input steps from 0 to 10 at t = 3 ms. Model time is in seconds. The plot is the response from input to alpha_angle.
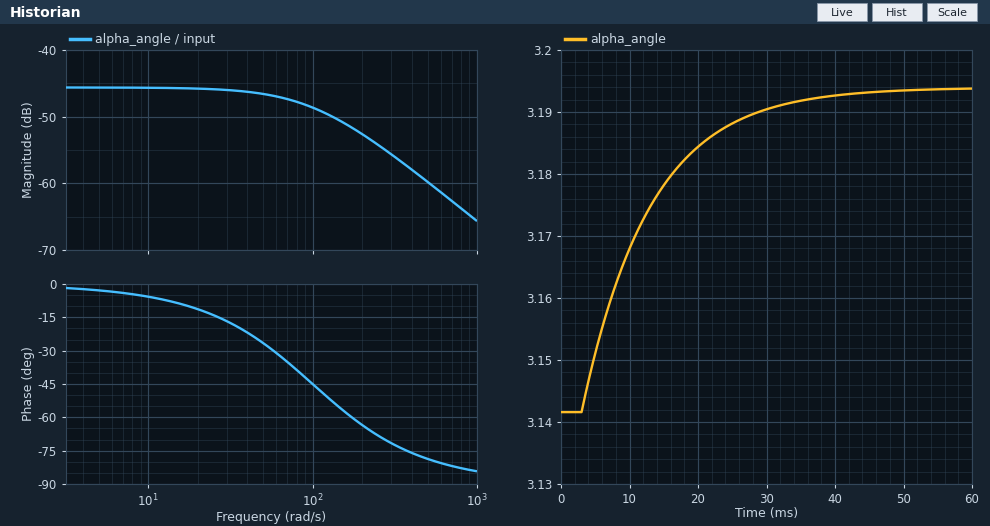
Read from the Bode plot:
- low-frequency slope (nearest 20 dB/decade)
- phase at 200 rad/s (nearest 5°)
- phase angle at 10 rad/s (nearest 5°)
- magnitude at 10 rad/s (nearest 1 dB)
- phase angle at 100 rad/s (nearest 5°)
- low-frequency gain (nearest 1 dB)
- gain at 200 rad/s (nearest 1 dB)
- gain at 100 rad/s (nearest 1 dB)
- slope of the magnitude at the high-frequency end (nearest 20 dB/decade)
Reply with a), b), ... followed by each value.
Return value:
a) 0 dB/decade
b) -65°
c) -5°
d) -46 dB
e) -45°
f) -46 dB
g) -53 dB
h) -49 dB
i) -20 dB/decade
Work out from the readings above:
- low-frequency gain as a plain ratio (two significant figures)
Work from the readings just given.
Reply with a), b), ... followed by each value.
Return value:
a) 0.0050
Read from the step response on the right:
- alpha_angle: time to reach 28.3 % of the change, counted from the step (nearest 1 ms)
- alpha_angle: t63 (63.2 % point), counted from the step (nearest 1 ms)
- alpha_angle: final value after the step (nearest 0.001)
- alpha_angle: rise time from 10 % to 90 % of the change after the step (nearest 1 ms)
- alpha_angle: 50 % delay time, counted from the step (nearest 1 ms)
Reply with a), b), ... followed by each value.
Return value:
a) 3 ms
b) 10 ms
c) 3.194
d) 22 ms
e) 7 ms
